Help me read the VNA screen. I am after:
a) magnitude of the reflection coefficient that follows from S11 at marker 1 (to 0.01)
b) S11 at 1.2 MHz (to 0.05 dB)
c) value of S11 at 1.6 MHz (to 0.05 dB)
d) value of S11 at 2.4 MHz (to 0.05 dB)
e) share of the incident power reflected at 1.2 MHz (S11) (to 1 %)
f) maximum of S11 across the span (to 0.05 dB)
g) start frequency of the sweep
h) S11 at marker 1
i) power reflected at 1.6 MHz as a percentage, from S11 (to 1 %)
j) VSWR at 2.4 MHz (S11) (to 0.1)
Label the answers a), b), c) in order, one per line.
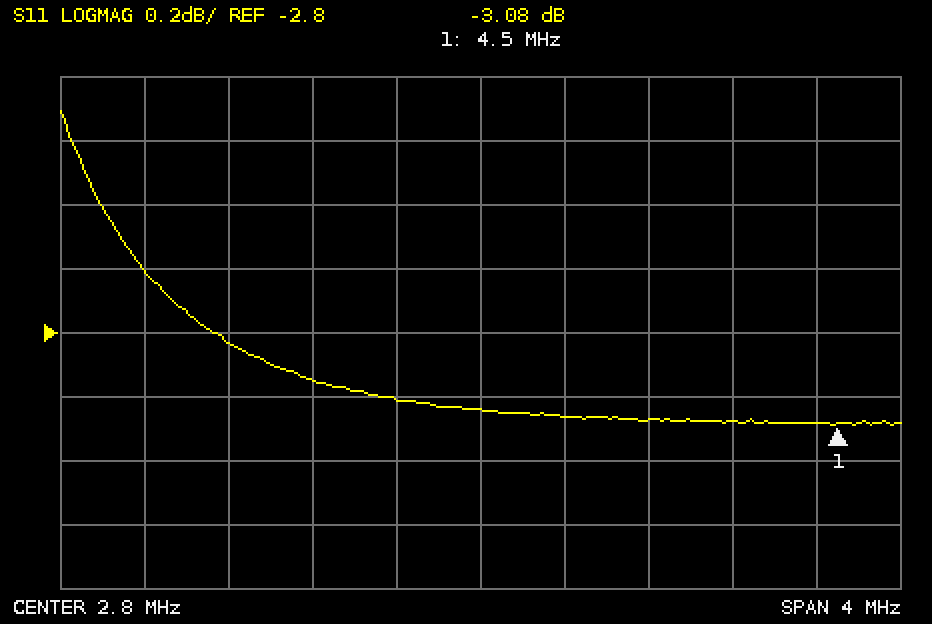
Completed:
a) 0.70
b) -2.60 dB
c) -2.85 dB
d) -3.00 dB
e) 55 %
f) -2.10 dB
g) 800 kHz
h) -3.08 dB
i) 52 %
j) 5.8
